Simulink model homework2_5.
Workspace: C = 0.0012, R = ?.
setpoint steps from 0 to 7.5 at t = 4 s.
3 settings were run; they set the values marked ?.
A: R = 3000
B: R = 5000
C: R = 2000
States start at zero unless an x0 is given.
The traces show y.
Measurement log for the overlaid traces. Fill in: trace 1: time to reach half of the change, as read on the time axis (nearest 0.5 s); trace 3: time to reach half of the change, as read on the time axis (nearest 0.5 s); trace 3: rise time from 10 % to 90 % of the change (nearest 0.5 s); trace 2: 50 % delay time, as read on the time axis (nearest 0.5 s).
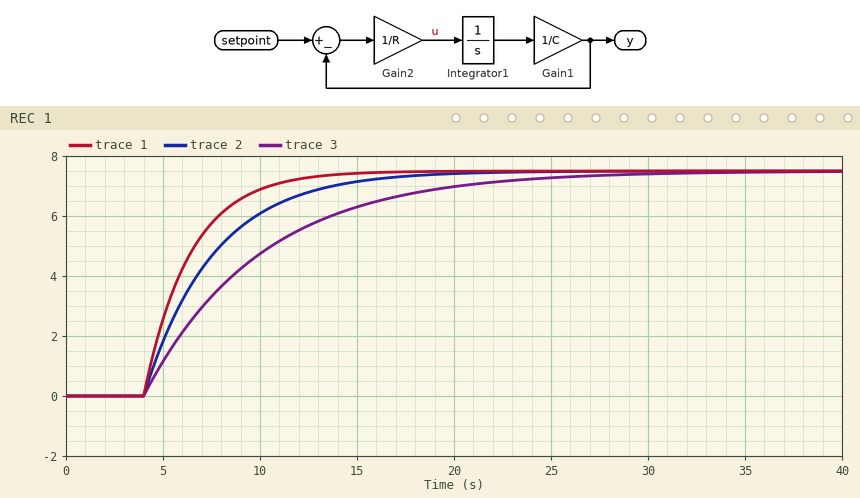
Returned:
5.5 s
8.0 s
13.0 s
6.5 s
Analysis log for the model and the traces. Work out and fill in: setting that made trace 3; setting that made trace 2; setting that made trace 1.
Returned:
B
A
C
